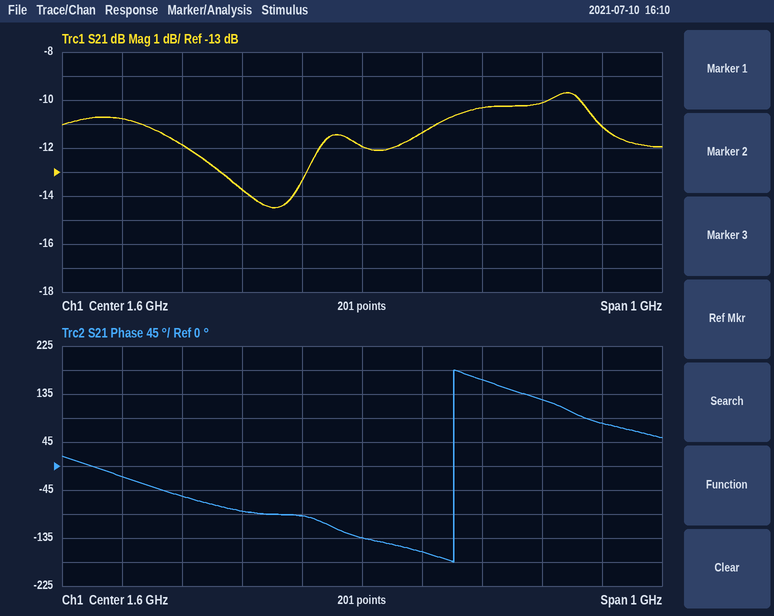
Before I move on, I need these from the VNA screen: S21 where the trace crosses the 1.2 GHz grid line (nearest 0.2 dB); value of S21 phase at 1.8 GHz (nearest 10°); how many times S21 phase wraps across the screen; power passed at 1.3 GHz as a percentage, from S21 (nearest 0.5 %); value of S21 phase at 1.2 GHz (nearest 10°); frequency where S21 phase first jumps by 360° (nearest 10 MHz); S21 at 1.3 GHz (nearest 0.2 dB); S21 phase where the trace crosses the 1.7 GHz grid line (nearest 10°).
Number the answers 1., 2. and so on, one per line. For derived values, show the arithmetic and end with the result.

1. -10.8 dB
2. 160°
3. 1
4. 10^(-11.8/10) ≈ 6.61 %, so 6.5 % to the nearest 0.5 %
5. -20°
6. 1.75 GHz
7. -11.8 dB
8. -160°
